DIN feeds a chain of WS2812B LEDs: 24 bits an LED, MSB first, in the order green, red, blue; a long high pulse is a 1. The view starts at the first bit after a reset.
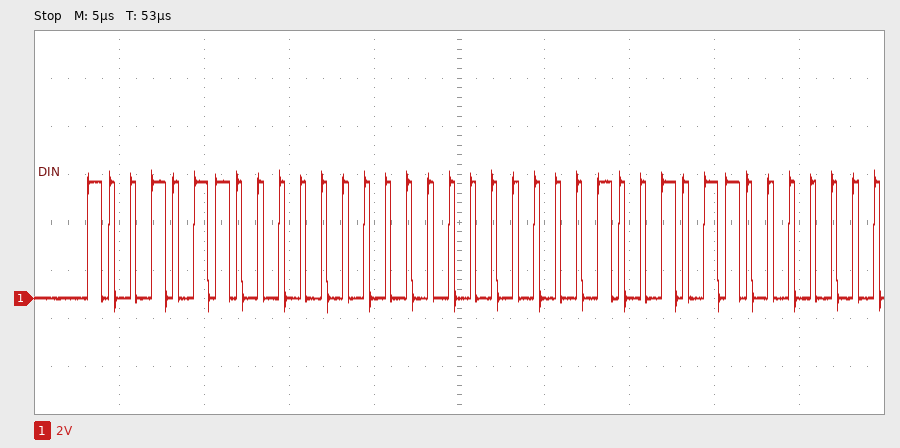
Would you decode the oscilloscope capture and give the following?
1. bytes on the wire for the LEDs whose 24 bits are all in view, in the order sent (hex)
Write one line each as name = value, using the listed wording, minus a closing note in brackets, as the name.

bytes on the wire for the LEDs whose 24 bits are all in view, in the order sent = 96 00 00
